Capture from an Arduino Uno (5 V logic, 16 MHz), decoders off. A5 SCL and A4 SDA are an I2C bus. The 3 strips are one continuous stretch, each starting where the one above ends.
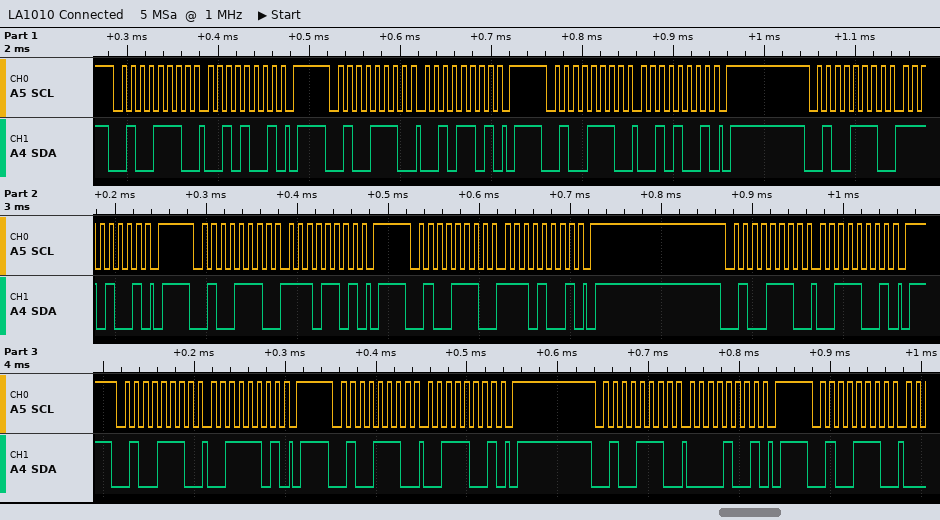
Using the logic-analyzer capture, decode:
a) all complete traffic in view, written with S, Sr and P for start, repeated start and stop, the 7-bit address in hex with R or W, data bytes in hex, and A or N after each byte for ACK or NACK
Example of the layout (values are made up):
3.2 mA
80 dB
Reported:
S 27W A 29 A P S 27W A 2D A P S 27W A 29 A P S 27W A E9 A P S 27W A ED A P S 27W A E9 A P S 27W A 39 A P S 27W A 3D A P S 27W A 39 A P S 27W A 09 A P S 27W A
